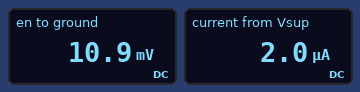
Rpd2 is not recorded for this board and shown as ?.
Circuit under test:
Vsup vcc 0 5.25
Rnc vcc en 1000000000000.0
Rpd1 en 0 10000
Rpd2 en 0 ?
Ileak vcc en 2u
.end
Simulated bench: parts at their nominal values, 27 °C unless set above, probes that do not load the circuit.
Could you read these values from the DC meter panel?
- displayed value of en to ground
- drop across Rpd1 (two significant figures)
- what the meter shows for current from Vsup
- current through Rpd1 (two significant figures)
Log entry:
10.9 mV
11 mV
2.0 µA
1.1 µA
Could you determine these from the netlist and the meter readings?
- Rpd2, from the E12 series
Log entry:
12 kΩ
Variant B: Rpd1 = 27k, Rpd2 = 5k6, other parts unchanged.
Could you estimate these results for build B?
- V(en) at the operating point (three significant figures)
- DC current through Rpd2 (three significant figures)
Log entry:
9.28 mV
1.66 µA
